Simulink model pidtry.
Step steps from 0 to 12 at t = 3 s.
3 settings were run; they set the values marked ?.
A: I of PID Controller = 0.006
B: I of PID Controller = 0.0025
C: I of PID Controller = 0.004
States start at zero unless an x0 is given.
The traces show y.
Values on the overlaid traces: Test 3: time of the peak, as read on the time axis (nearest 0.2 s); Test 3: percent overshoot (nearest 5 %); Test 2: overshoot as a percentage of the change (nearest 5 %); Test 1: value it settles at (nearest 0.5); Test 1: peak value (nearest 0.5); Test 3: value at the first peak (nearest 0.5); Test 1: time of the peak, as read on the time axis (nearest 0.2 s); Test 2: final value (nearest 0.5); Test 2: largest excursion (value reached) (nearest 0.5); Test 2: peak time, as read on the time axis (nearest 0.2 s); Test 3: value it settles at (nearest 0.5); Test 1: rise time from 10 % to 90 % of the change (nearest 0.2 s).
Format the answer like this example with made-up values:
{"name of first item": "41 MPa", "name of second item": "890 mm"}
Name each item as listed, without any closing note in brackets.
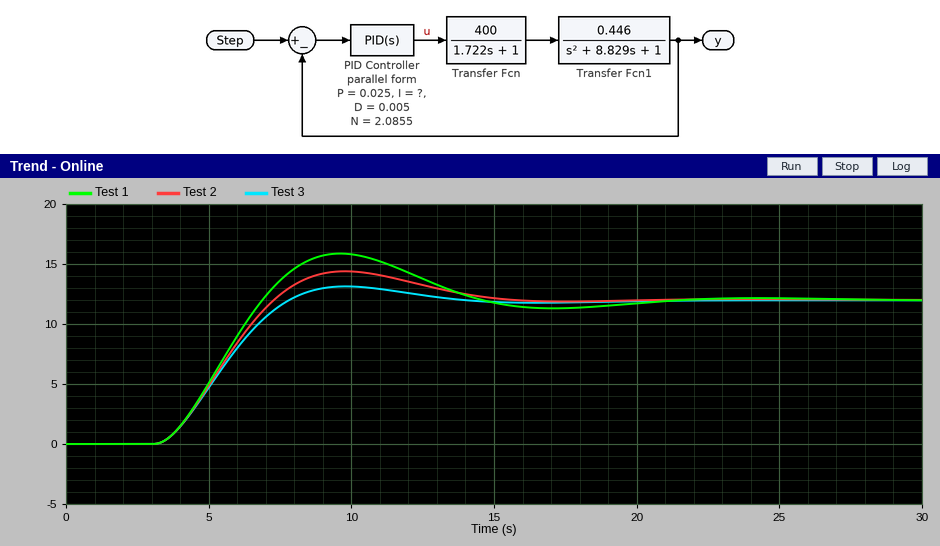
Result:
{"Test 3: time of the peak, as read on the time axis": "9.8 s", "Test 3: percent overshoot": "10 %", "Test 2: overshoot as a percentage of the change": "20 %", "Test 1: value it settles at": "12.0", "Test 1: peak value": "16.0", "Test 3: value at the first peak": "13.0", "Test 1: time of the peak, as read on the time axis": "9.6 s", "Test 2: final value": "12.0", "Test 2: largest excursion (value reached)": "14.5", "Test 2: peak time, as read on the time axis": "9.8 s", "Test 3: value it settles at": "12.0", "Test 1: rise time from 10 % to 90 % of the change": "2.6 s"}
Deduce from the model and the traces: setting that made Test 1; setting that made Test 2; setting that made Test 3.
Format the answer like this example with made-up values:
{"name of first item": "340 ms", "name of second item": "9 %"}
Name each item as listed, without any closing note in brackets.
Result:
{"setting that made Test 1": "A", "setting that made Test 2": "C", "setting that made Test 3": "B"}
